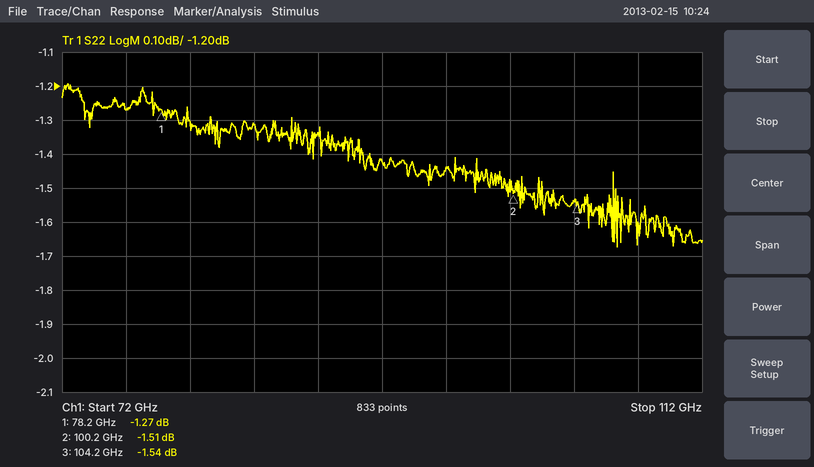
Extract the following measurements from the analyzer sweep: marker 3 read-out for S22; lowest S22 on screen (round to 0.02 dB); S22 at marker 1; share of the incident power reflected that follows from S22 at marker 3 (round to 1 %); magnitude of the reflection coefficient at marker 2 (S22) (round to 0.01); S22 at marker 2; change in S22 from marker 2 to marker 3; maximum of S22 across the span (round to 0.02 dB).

-1.54 dB
-1.68 dB
-1.27 dB
70 %
0.84
-1.51 dB
-0.03 dB
-1.20 dB
